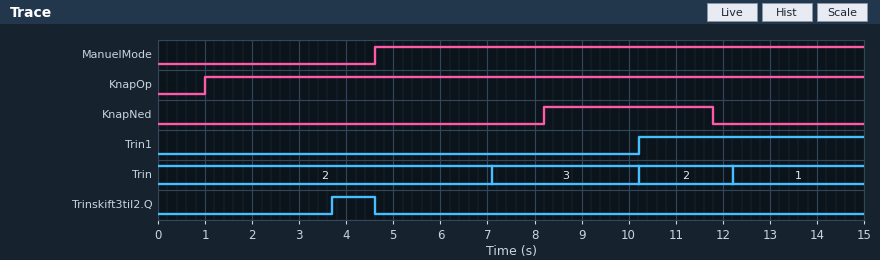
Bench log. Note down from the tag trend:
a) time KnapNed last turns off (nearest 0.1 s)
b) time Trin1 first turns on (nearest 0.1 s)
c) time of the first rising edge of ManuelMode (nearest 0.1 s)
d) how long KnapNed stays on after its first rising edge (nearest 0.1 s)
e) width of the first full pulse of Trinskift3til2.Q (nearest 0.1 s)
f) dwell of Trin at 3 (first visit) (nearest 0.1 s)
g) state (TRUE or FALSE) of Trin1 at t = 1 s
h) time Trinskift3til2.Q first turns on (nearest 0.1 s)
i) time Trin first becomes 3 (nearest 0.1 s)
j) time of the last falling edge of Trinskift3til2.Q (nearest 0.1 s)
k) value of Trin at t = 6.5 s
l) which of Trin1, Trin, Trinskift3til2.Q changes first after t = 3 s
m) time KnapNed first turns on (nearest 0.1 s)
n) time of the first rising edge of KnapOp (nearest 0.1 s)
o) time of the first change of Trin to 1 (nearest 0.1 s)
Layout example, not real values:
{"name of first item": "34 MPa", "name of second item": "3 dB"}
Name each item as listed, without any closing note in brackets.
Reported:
{"time KnapNed last turns off": "11.8 s", "time Trin1 first turns on": "10.2 s", "time of the first rising edge of ManuelMode": "4.6 s", "how long KnapNed stays on after its first rising edge": "3.6 s", "width of the first full pulse of Trinskift3til2.Q": "0.9 s", "dwell of Trin at 3 (first visit)": "3.1 s", "state (TRUE or FALSE) of Trin1 at t = 1 s": "FALSE", "time Trinskift3til2.Q first turns on": "3.7 s", "time Trin first becomes 3": "7.1 s", "time of the last falling edge of Trinskift3til2.Q": "4.6 s", "value of Trin at t = 6.5 s": "2", "which of Trin1, Trin, Trinskift3til2.Q changes first after t = 3 s": "Trinskift3til2.Q", "time KnapNed first turns on": "8.2 s", "time of the first rising edge of KnapOp": "1.0 s", "time of the first change of Trin to 1": "12.2 s"}
